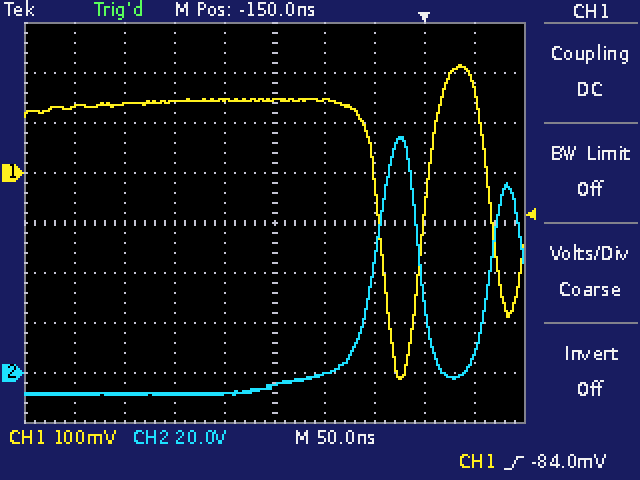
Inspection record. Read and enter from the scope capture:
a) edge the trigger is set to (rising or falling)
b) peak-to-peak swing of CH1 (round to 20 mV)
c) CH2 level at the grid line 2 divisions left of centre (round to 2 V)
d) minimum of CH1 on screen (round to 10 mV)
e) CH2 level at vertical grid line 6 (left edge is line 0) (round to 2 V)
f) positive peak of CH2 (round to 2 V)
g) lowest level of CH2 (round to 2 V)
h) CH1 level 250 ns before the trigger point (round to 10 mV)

rising
620 mV
-8 V
-410 mV
0 V
94 V
-8 V
140 mV
